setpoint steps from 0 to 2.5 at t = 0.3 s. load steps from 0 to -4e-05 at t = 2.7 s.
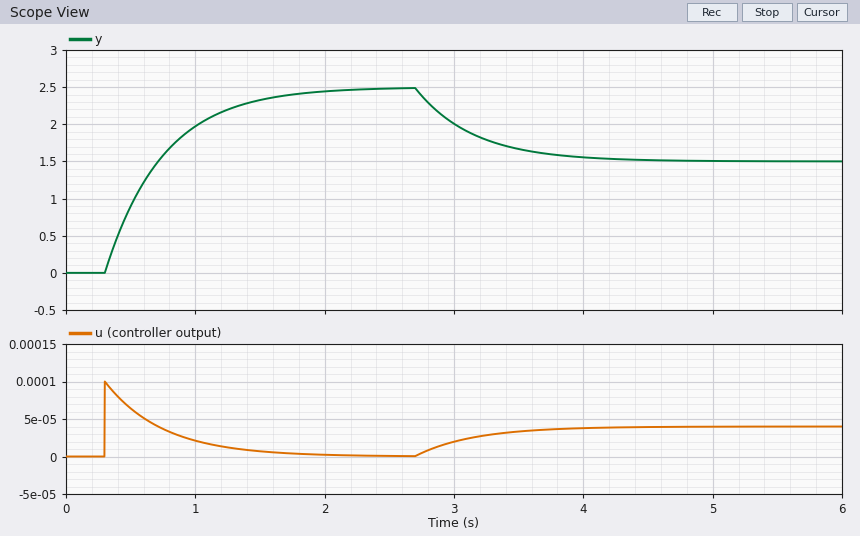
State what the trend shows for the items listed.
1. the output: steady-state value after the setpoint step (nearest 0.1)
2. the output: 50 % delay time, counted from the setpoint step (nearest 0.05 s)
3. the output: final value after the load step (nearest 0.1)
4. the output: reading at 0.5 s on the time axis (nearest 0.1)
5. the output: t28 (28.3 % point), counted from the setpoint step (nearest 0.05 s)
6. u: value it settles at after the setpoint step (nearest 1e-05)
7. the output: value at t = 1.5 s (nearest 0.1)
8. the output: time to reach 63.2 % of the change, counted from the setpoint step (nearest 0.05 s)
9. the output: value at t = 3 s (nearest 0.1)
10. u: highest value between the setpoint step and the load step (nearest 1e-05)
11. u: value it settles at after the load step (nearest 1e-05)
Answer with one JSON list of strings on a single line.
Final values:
["2.5", "0.30 s", "1.5", "0.9", "0.15 s", "0.00000", "2.3", "0.45 s", "2.0", "0.00010", "0.00004"]
